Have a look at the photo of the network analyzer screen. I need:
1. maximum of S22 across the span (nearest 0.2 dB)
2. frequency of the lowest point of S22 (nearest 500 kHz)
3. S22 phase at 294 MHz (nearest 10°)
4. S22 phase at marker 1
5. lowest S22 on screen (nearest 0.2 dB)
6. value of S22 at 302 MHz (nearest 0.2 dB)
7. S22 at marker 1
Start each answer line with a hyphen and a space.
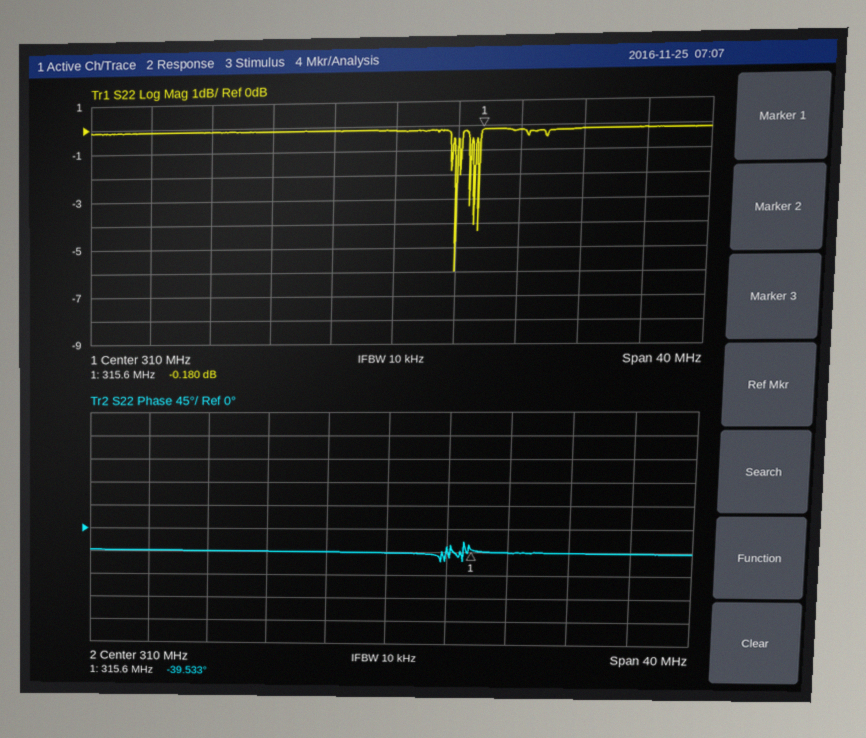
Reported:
- -0.2 dB
- 314.0 MHz
- -40°
- -39.533°
- -6.0 dB
- -0.2 dB
- -0.180 dB
